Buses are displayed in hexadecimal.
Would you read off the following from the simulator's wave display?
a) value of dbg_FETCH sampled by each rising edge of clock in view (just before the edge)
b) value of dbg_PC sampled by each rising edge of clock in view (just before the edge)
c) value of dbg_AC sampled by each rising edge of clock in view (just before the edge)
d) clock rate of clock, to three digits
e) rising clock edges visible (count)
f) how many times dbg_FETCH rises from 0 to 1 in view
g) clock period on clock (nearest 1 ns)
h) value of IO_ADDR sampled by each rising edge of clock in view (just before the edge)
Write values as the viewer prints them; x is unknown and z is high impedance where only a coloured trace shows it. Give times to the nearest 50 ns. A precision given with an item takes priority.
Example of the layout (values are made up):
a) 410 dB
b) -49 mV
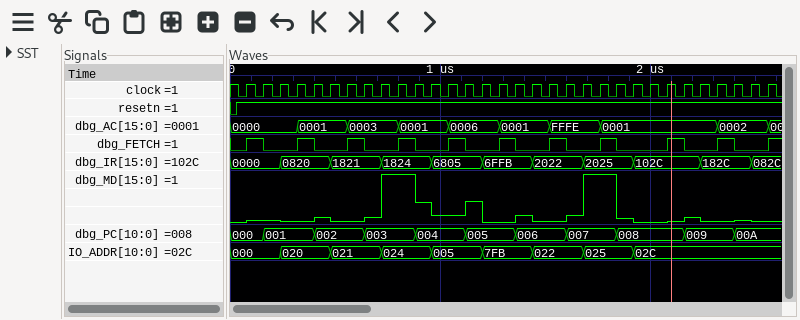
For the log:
a) 0 1 0 0 1 0 0 1 0 0 1 0 0 1 0 0 1 0 0 1 0 0 1 0 0 0 1 0 0 1 0 0
b) 000, 000, 001, 001, 001, 002, 002, 002, 003, 003, 003, 004, 004, 004, 005, 005, 005, 006, 006, 006, 007, 007, 007, 008, 008, 008, 008, 009, 009, 009, 00A, 00A
c) 0000, 0000, 0000, 0000, 0001, 0001, 0001, 0003, 0003, 0003, 0001, 0001, 0001, 0006, 0006, 0006, 0001, 0001, 0001, FFFE, FFFE, FFFE, 0001, 0001, 0001, 0001, 0001, 0001, 0001, 0002, 0002, 0002
d) 12.5 MHz
e) 32
f) 11
g) 80 ns
h) 000, 000, 000, 020, 020, 020, 021, 021, 021, 024, 024, 024, 005, 005, 005, 7FB, 7FB, 7FB, 022, 022, 022, 025, 025, 025, 02C, 02C, 02C, 02C, 02C, 02C, 02C, 02C
